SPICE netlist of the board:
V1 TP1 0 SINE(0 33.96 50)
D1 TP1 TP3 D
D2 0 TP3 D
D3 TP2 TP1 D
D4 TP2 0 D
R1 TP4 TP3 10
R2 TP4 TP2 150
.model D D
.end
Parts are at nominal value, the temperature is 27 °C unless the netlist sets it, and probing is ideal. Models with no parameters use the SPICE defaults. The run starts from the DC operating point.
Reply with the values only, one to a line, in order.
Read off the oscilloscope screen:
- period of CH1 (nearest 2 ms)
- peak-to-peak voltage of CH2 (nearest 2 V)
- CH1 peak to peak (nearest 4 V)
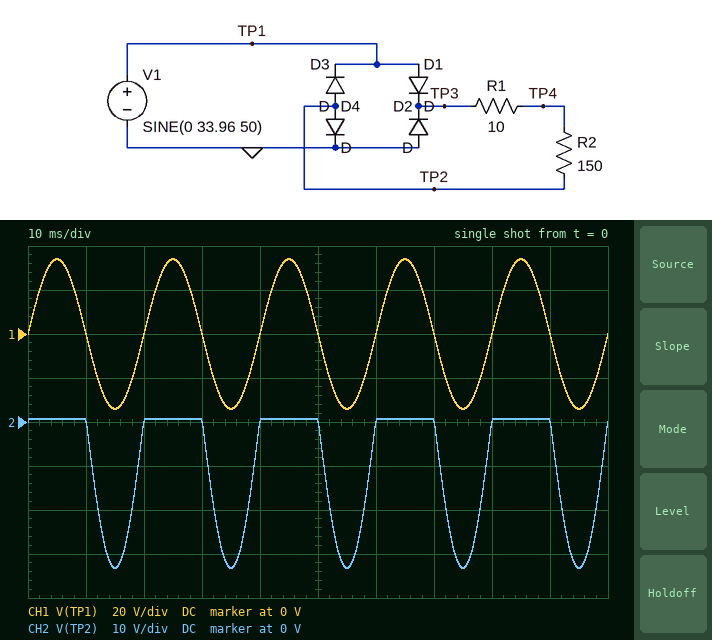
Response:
20 ms
34 V
68 V
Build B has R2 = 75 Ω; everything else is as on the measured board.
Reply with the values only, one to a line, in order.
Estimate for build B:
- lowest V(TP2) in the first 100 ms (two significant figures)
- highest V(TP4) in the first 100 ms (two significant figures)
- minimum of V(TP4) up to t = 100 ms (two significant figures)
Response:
-33 V
29 V
-4.6 V
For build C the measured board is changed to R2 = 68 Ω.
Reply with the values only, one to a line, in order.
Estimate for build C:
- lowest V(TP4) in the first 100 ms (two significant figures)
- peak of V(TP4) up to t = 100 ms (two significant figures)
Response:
-5.0 V
29 V
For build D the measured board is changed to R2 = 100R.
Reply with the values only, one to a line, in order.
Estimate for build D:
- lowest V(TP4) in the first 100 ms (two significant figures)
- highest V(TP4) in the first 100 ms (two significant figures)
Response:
-3.7 V
30 V
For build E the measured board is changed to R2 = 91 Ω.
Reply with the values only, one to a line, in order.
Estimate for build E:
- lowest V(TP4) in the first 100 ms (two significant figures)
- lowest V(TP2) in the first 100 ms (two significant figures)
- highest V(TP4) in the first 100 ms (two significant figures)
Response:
-4.0 V
-33 V
30 V
